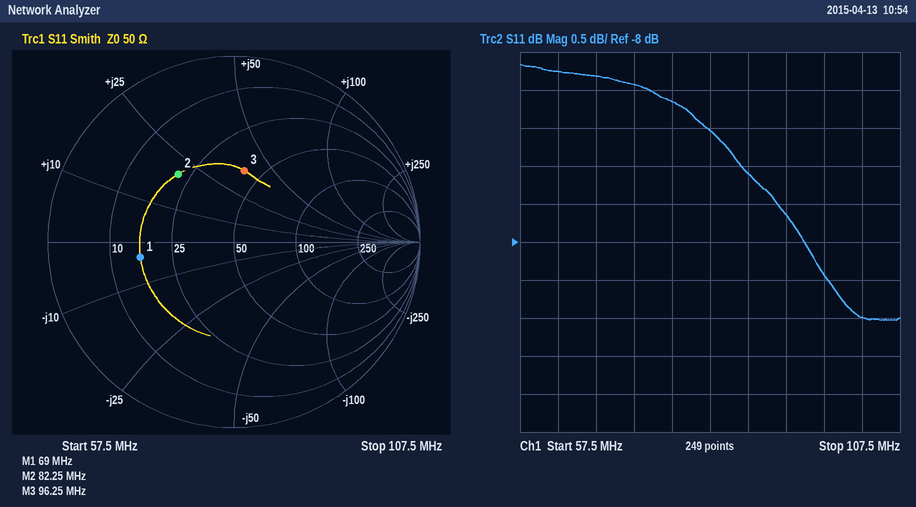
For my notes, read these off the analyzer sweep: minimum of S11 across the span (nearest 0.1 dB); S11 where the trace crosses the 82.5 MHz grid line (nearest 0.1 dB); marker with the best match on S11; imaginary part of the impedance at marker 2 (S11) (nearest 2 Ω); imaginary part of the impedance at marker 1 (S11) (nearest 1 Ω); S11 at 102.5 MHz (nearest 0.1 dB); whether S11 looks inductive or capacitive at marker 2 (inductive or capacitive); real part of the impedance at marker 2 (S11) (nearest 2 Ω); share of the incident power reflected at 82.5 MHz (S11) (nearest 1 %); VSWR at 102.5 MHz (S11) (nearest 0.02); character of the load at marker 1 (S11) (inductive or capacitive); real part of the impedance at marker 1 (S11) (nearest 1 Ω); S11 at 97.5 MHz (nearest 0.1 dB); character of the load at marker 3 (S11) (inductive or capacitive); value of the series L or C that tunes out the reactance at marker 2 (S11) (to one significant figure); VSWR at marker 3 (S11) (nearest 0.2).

-9.0 dB
-6.5 dB
marker 3
+20 Ω
-4 Ω
-9.0 dB
inductive
22 Ω
22 %
2.10
capacitive
16 Ω
-8.4 dB
inductive
100 pF
2.2
